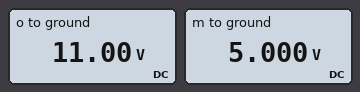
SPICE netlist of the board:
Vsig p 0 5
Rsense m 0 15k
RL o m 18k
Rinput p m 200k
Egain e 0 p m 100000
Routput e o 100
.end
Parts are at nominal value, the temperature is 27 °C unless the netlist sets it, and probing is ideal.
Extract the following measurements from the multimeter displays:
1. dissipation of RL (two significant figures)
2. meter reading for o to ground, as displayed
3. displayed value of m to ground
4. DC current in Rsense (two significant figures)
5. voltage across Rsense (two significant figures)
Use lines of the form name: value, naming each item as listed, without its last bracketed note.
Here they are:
dissipation of RL: 2.0 mW
meter reading for o to ground, as displayed: 11.00 V
displayed value of m to ground: 5.000 V
DC current in Rsense: 330 µA
voltage across Rsense: 5.0 V
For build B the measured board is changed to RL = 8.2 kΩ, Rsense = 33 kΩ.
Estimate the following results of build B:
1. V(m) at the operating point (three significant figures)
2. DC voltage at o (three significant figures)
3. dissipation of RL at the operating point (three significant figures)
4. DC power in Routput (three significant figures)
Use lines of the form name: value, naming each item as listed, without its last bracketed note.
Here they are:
V(m) at the operating point: 5.00 V
DC voltage at o: 6.24 V
dissipation of RL at the operating point: 188 µW
DC power in Routput: 2.30 µW
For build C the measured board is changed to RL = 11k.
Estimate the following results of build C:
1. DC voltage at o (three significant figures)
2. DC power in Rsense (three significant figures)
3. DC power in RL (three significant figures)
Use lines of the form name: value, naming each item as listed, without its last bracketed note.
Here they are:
DC voltage at o: 8.67 V
DC power in Rsense: 1.67 mW
DC power in RL: 1.22 mW
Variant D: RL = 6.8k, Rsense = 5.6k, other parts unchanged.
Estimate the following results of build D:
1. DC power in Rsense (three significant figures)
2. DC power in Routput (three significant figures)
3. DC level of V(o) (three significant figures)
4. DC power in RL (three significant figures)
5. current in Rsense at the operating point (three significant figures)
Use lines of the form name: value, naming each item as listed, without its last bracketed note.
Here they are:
DC power in Rsense: 4.46 mW
DC power in Routput: 79.7 µW
DC level of V(o): 11.1 V
DC power in RL: 5.42 mW
current in Rsense at the operating point: 893 µA
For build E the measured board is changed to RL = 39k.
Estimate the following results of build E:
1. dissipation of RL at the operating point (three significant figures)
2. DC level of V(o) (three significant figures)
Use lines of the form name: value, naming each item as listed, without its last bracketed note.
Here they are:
dissipation of RL at the operating point: 4.33 mW
DC level of V(o): 18.0 V
